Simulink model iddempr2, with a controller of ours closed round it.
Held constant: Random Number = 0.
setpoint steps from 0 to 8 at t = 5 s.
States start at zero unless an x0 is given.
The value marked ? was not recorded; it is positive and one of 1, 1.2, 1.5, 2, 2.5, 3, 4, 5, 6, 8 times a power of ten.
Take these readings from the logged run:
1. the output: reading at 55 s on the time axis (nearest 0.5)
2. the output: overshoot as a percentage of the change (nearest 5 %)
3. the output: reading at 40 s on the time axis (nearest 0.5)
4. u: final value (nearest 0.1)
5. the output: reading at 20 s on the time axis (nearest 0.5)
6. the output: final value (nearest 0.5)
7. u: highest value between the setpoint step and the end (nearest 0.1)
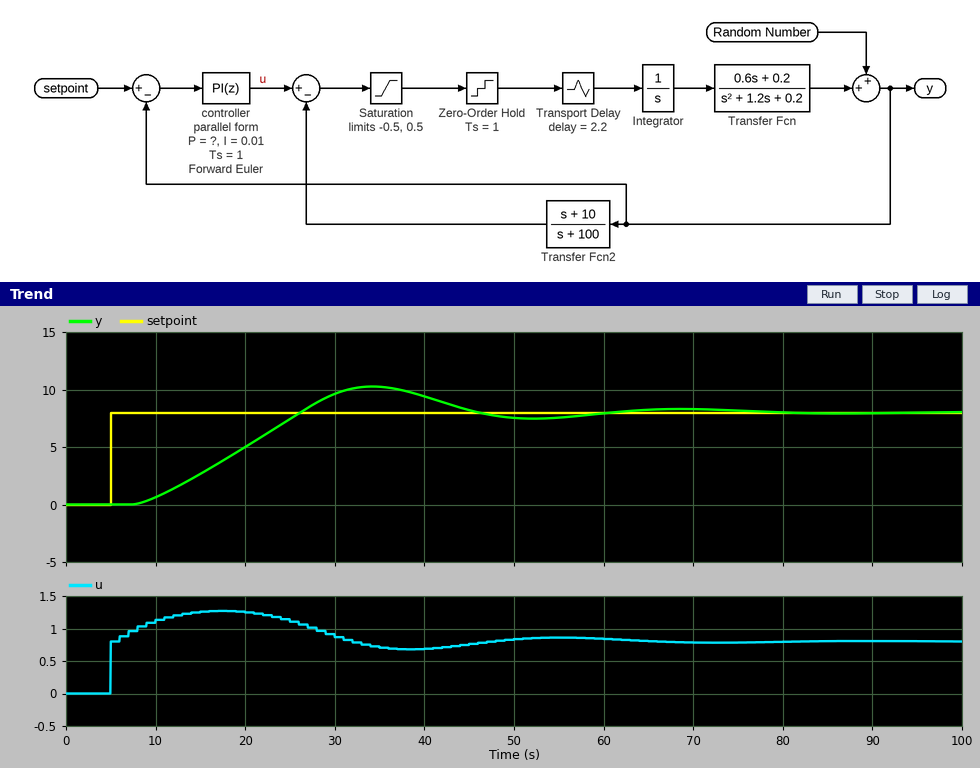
7.5
30 %
9.5
0.8
5.0
8.0
1.3
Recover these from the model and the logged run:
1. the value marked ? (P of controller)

0.1
